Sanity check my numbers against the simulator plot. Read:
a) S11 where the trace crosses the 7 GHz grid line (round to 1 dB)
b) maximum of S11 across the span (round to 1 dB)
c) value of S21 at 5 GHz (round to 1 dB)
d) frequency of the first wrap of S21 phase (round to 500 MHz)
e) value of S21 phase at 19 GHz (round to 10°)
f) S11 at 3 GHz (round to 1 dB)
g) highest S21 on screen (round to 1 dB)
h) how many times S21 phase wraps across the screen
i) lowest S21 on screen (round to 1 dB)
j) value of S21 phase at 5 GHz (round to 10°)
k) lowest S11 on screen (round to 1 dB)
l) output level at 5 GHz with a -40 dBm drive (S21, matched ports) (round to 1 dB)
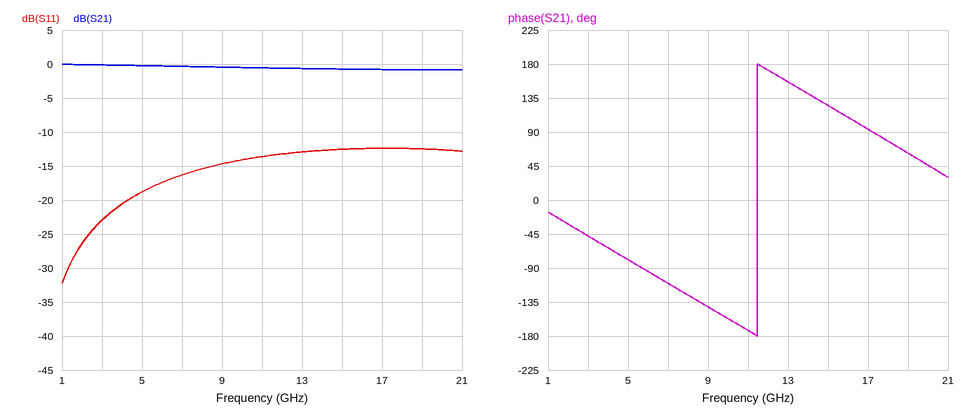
-16 dB
-12 dB
0 dB
11.5 GHz
60°
-23 dB
0 dB
1
-1 dB
-80°
-32 dB
-40 dBm
